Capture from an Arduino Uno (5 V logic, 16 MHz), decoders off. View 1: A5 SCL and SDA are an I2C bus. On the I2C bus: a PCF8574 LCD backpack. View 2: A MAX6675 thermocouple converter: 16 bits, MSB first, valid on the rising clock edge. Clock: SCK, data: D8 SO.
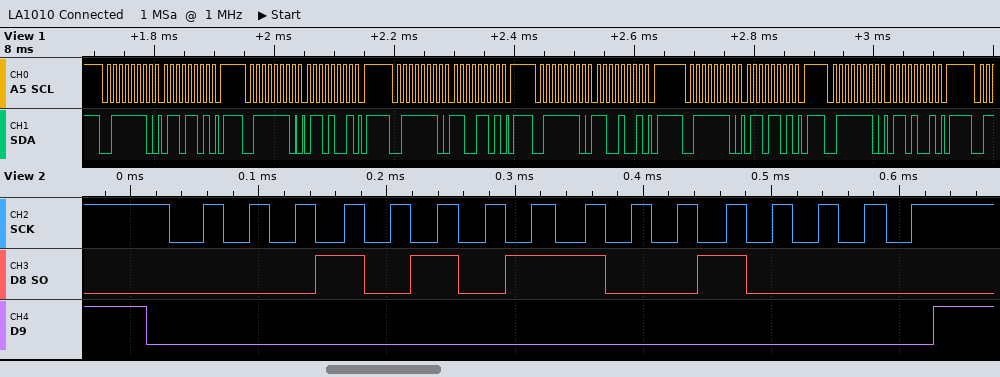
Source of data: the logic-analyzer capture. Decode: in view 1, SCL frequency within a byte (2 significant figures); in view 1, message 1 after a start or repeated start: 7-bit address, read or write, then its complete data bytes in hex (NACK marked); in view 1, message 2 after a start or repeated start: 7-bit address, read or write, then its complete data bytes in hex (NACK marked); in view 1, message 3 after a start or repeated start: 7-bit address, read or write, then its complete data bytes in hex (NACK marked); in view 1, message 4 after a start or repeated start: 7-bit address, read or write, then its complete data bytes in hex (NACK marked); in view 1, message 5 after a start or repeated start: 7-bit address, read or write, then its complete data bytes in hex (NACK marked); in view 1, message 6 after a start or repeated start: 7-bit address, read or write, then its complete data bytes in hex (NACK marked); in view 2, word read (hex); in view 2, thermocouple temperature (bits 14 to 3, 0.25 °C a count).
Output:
100 kHz
0x3F write: 6D
0x3F write: 69
0x3F write: CD
0x3F write: C9
0x3F write: 6D
0x3F write: 69
0x1590
172.50 °C
